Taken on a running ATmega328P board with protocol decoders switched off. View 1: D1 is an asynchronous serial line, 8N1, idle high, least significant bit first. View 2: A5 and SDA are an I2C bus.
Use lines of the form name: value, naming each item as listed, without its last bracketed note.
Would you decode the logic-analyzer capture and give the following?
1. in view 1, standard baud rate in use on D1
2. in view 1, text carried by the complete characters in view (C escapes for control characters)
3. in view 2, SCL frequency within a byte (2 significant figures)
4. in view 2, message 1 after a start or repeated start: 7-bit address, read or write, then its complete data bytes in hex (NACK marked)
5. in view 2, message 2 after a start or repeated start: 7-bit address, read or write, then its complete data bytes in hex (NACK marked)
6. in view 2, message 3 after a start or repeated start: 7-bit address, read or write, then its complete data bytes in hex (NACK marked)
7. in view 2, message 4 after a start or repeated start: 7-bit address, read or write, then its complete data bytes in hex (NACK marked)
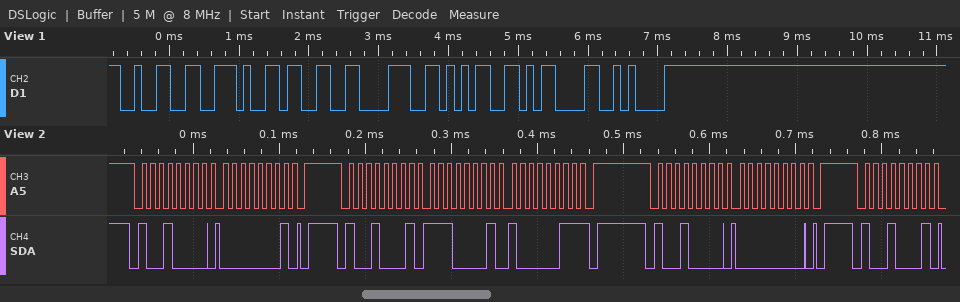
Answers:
in view 1, standard baud rate in use on D1: 9600 baud
in view 1, text carried by the complete characters in view: "2.385\r\n"
in view 2, SCL frequency within a byte: 100 kHz
in view 2, message 1 after a start or repeated start: 7-bit address, read or write, then its complete data bytes in hex: 0x48 write: 01
in view 2, message 2 after a start or repeated start: 7-bit address, read or write, then its complete data bytes in hex: 0x48 read: E1 83 NACK
in view 2, message 3 after a start or repeated start: 7-bit address, read or write, then its complete data bytes in hex: 0x48 write: 00
in view 2, message 4 after a start or repeated start: 7-bit address, read or write, then its complete data bytes in hex: 0x48 read
